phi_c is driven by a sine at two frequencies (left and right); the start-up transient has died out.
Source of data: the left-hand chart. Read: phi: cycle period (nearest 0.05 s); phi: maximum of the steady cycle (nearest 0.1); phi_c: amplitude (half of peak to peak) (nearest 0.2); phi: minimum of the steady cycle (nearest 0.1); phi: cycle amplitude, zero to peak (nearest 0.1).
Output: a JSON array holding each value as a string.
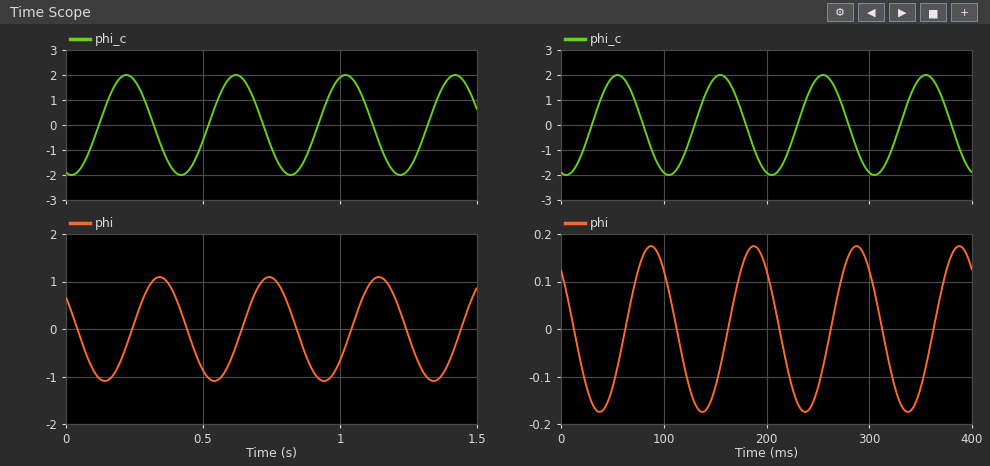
["0.40 s", "1.1", "2.0", "-1.1", "1.1"]
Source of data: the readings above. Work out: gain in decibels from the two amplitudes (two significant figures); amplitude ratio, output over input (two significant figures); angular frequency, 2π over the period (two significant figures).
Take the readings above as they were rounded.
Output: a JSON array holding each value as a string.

["-5.2 dB", "0.55", "16 rad/s"]
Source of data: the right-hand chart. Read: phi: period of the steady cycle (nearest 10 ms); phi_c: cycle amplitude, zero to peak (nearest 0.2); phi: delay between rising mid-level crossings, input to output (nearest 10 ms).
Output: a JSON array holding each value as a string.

["100 ms", "2.0", "30 ms"]
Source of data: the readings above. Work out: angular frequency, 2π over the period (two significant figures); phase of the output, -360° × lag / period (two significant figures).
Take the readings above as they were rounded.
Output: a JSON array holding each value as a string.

["0.063 rad/ms", "-110°"]
